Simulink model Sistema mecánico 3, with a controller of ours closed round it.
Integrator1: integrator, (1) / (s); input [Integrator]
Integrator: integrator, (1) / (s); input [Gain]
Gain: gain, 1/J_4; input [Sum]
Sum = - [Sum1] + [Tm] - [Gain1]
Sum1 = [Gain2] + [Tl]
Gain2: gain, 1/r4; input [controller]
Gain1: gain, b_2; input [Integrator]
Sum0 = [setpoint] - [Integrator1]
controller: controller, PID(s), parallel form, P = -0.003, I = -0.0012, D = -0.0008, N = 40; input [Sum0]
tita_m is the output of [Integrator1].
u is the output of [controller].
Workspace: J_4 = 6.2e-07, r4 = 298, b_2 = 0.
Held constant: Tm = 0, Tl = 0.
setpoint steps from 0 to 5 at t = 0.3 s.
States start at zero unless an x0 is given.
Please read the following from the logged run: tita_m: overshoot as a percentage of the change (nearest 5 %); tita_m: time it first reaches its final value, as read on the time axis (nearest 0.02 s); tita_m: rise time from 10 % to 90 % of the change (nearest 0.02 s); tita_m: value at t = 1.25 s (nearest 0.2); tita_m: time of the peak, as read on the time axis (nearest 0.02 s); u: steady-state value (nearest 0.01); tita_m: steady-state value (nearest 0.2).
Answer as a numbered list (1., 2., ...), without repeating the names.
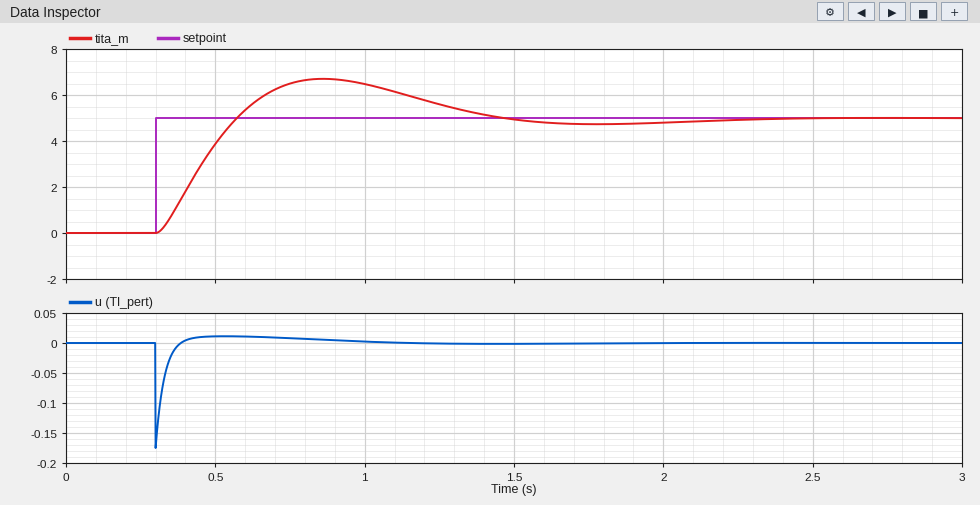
1. 35 %
2. 0.58 s
3. 0.20 s
4. 5.6
5. 0.86 s
6. 0.00
7. 5.0
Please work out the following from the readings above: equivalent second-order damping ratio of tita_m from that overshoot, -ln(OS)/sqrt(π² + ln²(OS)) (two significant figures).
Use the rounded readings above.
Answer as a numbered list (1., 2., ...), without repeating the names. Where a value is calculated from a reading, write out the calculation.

1. ln(0.35) = -1.050; 1.050 / sqrt(9.870 + 1.102) = 0.32
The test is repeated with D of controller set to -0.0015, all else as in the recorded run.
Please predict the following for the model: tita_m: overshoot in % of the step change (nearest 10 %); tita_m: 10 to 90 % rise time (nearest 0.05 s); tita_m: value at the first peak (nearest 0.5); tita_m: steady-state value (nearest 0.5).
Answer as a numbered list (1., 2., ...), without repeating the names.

1. 20 %
2. 0.15 s
3. 6.0
4. 5.0
